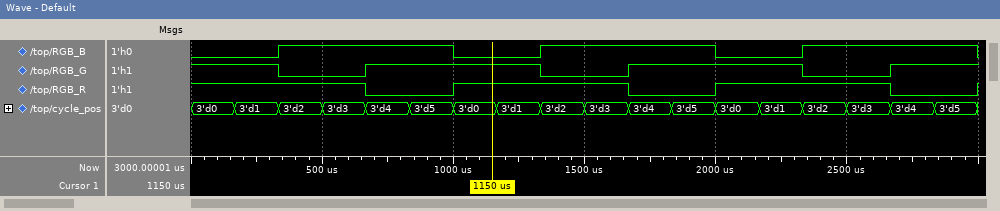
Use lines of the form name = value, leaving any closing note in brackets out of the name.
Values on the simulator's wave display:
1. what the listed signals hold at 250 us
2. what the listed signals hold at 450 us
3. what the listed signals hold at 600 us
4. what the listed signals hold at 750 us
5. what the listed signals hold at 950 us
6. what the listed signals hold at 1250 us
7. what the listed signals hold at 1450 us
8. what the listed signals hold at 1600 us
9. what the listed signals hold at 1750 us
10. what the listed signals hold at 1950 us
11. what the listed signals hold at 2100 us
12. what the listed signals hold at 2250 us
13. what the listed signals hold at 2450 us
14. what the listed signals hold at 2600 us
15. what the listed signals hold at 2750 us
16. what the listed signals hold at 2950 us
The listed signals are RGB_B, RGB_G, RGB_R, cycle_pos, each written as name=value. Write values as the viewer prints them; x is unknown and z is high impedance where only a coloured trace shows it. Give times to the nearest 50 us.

what the listed signals hold at 250 us = RGB_B=0, RGB_G=1, RGB_R=1, cycle_pos=3'd1
what the listed signals hold at 450 us = RGB_B=1, RGB_G=0, RGB_R=1, cycle_pos=3'd2
what the listed signals hold at 600 us = RGB_B=1, RGB_G=0, RGB_R=1, cycle_pos=3'd3
what the listed signals hold at 750 us = RGB_B=1, RGB_G=1, RGB_R=0, cycle_pos=3'd4
what the listed signals hold at 950 us = RGB_B=1, RGB_G=1, RGB_R=0, cycle_pos=3'd5
what the listed signals hold at 1250 us = RGB_B=0, RGB_G=1, RGB_R=1, cycle_pos=3'd1
what the listed signals hold at 1450 us = RGB_B=1, RGB_G=0, RGB_R=1, cycle_pos=3'd2
what the listed signals hold at 1600 us = RGB_B=1, RGB_G=0, RGB_R=1, cycle_pos=3'd3
what the listed signals hold at 1750 us = RGB_B=1, RGB_G=1, RGB_R=0, cycle_pos=3'd4
what the listed signals hold at 1950 us = RGB_B=1, RGB_G=1, RGB_R=0, cycle_pos=3'd5
what the listed signals hold at 2100 us = RGB_B=0, RGB_G=1, RGB_R=1, cycle_pos=3'd0
what the listed signals hold at 2250 us = RGB_B=0, RGB_G=1, RGB_R=1, cycle_pos=3'd1
what the listed signals hold at 2450 us = RGB_B=1, RGB_G=0, RGB_R=1, cycle_pos=3'd2
what the listed signals hold at 2600 us = RGB_B=1, RGB_G=0, RGB_R=1, cycle_pos=3'd3
what the listed signals hold at 2750 us = RGB_B=1, RGB_G=1, RGB_R=0, cycle_pos=3'd4
what the listed signals hold at 2950 us = RGB_B=1, RGB_G=1, RGB_R=0, cycle_pos=3'd5
